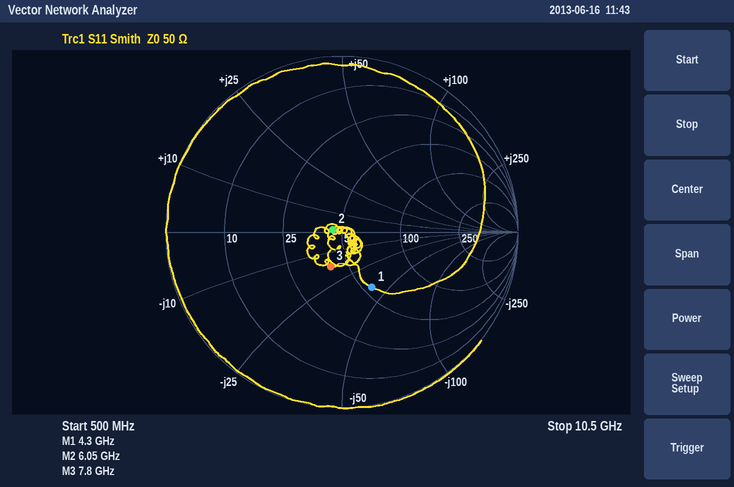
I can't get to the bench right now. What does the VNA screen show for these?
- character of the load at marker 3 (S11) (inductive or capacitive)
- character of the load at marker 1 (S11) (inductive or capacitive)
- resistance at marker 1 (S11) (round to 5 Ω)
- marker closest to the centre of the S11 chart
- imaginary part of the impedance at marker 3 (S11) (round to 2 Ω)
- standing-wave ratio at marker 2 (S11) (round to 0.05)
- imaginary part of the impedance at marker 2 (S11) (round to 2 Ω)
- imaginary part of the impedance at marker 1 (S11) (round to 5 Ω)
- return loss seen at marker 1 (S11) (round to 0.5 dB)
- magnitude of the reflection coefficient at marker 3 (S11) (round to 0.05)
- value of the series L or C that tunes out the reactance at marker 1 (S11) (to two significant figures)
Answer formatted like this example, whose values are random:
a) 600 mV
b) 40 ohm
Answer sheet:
a) capacitive
b) capacitive
c) 55 Ω
d) marker 2
e) -16 Ω
f) 1.10
g) +2 Ω
h) -40 Ω
i) 9.0 dB
j) 0.20
k) 1.5 nH
